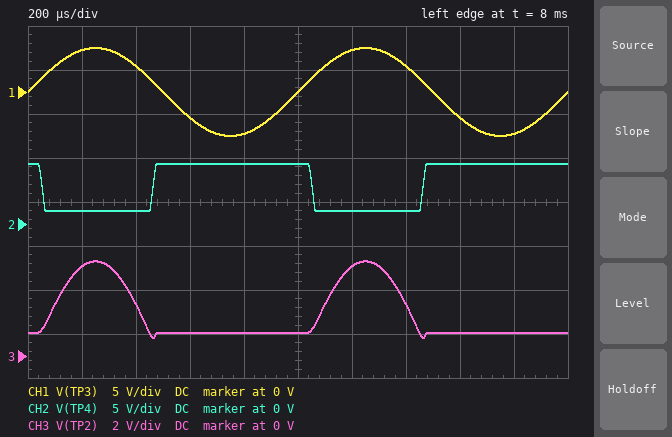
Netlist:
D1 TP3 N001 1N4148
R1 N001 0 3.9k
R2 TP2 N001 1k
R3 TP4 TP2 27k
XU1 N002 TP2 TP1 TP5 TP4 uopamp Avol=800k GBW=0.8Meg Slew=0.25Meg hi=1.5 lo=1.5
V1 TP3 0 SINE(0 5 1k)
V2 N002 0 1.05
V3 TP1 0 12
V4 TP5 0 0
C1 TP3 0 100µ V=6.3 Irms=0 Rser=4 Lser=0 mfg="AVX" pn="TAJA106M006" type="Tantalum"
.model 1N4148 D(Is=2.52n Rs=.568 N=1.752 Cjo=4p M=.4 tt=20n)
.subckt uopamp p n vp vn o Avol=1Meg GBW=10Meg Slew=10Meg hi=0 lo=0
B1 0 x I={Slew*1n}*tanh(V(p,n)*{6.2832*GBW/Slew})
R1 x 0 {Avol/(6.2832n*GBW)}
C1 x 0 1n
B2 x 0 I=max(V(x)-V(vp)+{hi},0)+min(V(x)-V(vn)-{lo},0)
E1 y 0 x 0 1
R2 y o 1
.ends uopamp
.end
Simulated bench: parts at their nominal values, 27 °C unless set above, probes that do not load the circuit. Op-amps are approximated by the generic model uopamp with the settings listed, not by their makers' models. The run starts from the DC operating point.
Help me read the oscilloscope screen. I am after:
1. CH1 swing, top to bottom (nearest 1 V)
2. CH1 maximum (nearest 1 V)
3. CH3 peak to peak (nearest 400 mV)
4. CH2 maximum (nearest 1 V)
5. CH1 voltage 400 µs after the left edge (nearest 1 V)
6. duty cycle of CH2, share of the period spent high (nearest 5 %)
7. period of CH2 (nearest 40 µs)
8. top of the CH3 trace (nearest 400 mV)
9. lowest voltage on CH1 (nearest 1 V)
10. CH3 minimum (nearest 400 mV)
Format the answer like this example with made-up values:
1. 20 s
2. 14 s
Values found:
1. 10 V
2. 5 V
3. 3.6 V
4. 7 V
5. 3 V
6. 60 %
7. 1.00 ms
8. 4.4 V
9. -5 V
10. 800 mV
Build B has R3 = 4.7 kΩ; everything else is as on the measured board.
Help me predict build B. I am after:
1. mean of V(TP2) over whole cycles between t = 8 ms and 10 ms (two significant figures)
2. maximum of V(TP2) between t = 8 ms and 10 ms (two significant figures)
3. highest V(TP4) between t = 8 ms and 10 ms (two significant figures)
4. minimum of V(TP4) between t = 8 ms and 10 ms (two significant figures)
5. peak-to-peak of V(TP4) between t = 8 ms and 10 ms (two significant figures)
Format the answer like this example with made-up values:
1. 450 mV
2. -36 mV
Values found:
1. 1.8 V
2. 3.9 V
3. 2.1 V
4. 1.5 V
5. 560 mV
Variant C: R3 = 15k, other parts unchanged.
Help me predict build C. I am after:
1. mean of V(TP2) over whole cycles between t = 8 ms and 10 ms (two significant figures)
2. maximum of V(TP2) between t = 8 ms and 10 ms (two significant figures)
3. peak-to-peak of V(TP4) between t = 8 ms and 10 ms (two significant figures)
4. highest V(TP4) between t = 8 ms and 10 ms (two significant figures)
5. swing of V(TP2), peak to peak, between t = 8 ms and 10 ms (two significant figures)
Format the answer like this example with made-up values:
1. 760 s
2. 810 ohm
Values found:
1. 1.9 V
2. 4.2 V
3. 2.8 V
4. 4.3 V
5. 3.3 V
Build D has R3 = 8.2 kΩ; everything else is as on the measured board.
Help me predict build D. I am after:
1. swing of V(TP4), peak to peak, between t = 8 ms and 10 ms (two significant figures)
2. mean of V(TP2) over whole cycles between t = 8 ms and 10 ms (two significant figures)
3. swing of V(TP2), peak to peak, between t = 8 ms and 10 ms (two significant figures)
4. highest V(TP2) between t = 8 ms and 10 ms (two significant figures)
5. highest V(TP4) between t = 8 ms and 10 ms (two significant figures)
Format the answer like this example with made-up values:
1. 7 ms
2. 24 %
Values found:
1. 1.3 V
2. 1.8 V
3. 3.1 V
4. 4.1 V
5. 2.8 V
